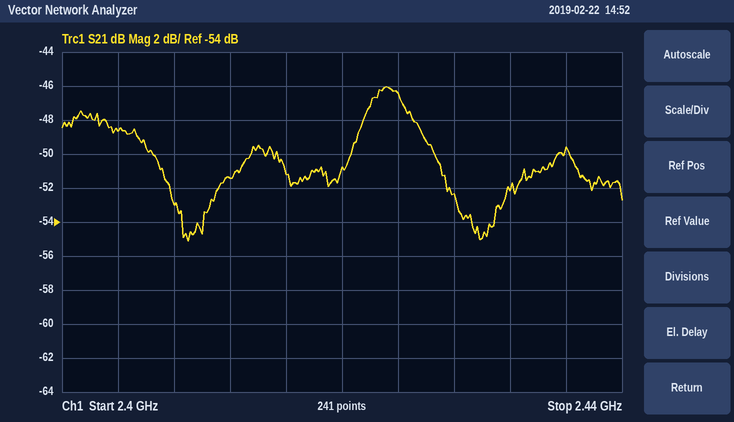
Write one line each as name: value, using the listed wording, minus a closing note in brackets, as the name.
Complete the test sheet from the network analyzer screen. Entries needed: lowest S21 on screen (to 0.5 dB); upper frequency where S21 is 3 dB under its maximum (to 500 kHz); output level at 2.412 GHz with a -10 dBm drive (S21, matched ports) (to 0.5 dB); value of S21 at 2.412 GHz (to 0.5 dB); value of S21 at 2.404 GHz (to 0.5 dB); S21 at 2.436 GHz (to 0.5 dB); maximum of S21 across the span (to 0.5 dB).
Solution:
lowest S21 on screen: -55.0 dB
upper frequency where S21 is 3 dB under its maximum: 2.4260 GHz
output level at 2.412 GHz with a -10 dBm drive (S21, matched ports): -61.5 dBm
value of S21 at 2.412 GHz: -51.5 dB
value of S21 at 2.404 GHz: -48.5 dB
S21 at 2.436 GHz: -49.5 dB
maximum of S21 across the span: -46.0 dB
